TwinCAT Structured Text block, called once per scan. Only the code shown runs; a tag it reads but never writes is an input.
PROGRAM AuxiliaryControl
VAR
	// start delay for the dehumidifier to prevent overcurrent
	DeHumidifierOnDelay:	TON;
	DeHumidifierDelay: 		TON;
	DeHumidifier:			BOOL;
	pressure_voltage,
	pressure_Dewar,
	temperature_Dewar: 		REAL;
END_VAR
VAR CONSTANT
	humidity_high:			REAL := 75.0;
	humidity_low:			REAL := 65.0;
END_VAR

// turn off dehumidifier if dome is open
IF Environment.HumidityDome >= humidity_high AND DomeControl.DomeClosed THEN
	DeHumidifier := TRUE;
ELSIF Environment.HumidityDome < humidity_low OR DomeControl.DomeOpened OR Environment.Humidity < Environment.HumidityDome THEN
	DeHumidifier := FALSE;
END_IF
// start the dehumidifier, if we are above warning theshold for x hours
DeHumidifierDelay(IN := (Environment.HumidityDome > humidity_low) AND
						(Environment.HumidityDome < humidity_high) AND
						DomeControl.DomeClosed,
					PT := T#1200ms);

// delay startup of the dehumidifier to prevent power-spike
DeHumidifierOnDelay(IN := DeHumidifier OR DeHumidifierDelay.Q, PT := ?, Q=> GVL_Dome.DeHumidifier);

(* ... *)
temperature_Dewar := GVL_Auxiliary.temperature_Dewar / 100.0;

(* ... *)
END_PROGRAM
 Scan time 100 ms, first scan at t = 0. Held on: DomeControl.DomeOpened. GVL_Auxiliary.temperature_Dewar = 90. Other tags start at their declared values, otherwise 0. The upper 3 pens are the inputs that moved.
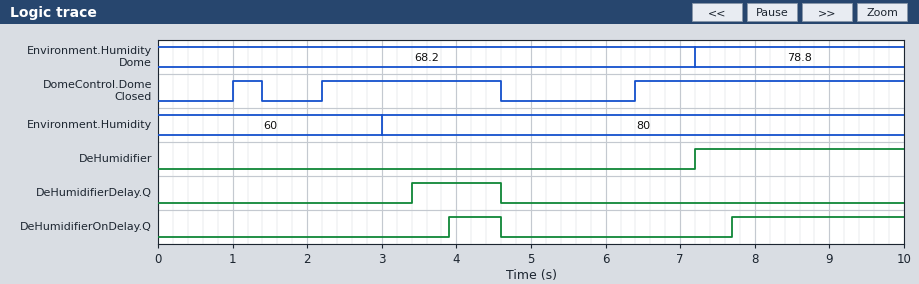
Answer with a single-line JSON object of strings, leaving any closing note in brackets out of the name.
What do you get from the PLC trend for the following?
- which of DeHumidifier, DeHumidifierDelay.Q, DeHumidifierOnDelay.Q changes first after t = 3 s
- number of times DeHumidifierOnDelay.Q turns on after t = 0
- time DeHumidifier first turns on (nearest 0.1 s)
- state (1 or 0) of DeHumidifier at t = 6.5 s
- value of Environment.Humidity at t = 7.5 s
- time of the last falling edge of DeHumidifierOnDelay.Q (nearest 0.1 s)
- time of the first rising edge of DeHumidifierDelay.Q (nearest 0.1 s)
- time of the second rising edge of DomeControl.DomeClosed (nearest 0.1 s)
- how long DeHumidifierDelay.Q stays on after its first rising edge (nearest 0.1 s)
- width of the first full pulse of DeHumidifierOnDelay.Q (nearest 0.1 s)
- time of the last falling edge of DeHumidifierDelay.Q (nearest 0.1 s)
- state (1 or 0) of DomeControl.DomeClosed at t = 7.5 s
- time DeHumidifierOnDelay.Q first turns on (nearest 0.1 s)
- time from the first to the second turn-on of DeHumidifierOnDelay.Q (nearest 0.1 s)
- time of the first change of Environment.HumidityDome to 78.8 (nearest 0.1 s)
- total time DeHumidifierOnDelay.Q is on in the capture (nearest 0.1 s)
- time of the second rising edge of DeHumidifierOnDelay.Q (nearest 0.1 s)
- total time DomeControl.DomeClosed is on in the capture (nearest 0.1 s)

{"which of DeHumidifier, DeHumidifierDelay.Q, DeHumidifierOnDelay.Q changes first after t = 3 s": "DeHumidifierDelay.Q", "number of times DeHumidifierOnDelay.Q turns on after t = 0": "2", "time DeHumidifier first turns on": "7.2 s", "state (1 or 0) of DeHumidifier at t = 6.5 s": "0", "value of Environment.Humidity at t = 7.5 s": "80", "time of the last falling edge of DeHumidifierOnDelay.Q": "4.6 s", "time of the first rising edge of DeHumidifierDelay.Q": "3.4 s", "time of the second rising edge of DomeControl.DomeClosed": "2.2 s", "how long DeHumidifierDelay.Q stays on after its first rising edge": "1.2 s", "width of the first full pulse of DeHumidifierOnDelay.Q": "0.7 s", "time of the last falling edge of DeHumidifierDelay.Q": "4.6 s", "state (1 or 0) of DomeControl.DomeClosed at t = 7.5 s": "1", "time DeHumidifierOnDelay.Q first turns on": "3.9 s", "time from the first to the second turn-on of DeHumidifierOnDelay.Q": "3.8 s", "time of the first change of Environment.HumidityDome to 78.8": "7.2 s", "total time DeHumidifierOnDelay.Q is on in the capture": "3.0 s", "time of the second rising edge of DeHumidifierOnDelay.Q": "7.7 s", "total time DomeControl.DomeClosed is on in the capture": "6.4 s"}
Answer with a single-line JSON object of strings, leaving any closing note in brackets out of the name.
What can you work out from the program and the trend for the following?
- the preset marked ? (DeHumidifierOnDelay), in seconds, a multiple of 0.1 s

{"the preset marked ? (DeHumidifierOnDelay), in seconds, a multiple of 0.1 s": "0.5 s"}
